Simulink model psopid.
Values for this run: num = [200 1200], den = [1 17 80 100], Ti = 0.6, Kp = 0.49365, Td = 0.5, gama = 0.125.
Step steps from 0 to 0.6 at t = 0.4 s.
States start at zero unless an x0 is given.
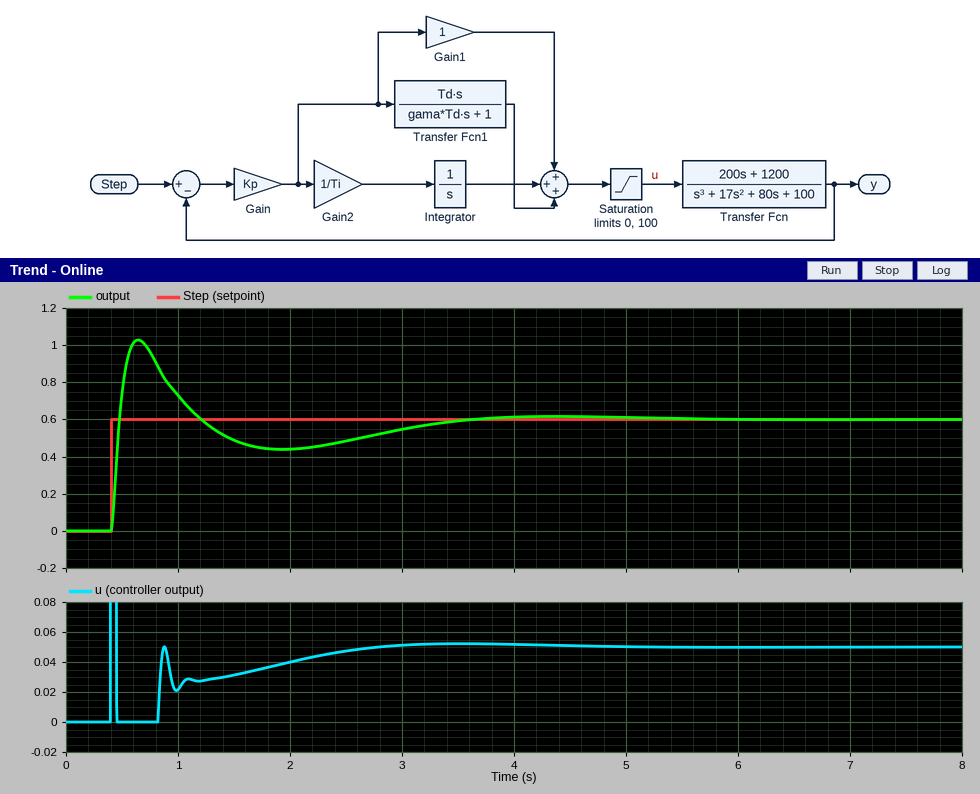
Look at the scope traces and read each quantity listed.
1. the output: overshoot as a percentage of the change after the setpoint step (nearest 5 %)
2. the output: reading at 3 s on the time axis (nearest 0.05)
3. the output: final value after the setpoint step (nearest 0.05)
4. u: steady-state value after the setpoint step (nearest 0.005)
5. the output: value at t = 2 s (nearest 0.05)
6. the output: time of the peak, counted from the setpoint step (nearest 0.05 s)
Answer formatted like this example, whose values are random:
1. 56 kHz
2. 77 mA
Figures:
1. 70 %
2. 0.55
3. 0.60
4. 0.050
5. 0.45
6. 0.25 s
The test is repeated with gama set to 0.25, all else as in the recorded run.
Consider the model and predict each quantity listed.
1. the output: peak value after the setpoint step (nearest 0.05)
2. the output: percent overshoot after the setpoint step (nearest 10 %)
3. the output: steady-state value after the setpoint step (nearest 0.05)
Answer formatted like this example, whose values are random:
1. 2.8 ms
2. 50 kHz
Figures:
1. 0.90
2. 50 %
3. 0.60
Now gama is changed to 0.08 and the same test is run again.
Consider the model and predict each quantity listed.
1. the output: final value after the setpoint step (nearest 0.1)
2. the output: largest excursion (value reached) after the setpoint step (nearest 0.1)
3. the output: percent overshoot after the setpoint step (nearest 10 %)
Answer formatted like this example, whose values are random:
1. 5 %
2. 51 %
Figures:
1. 0.6
2. 1.1
3. 90 %
